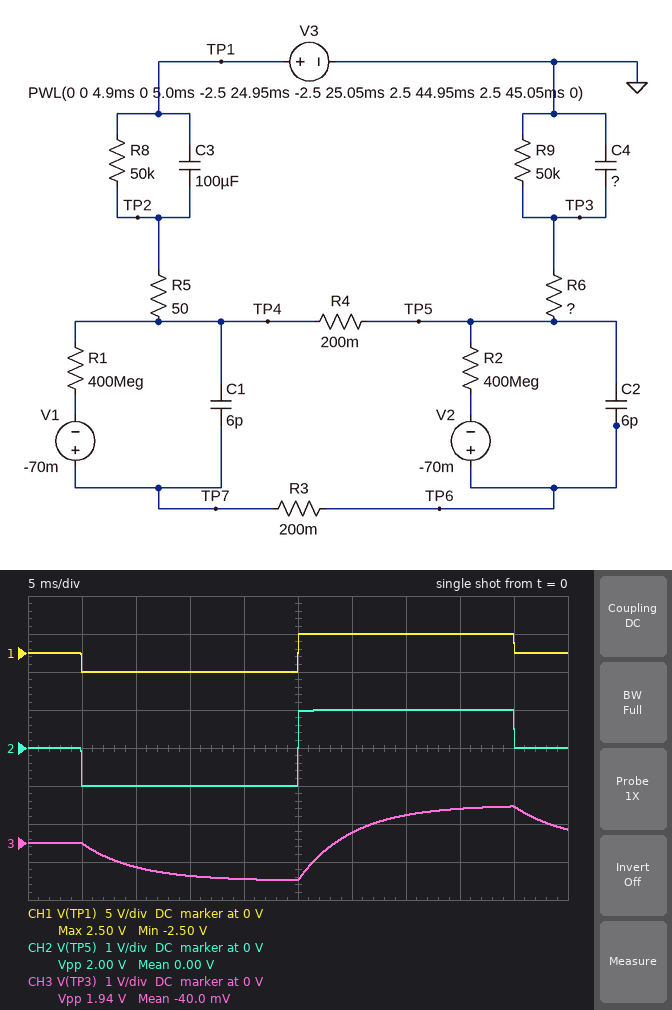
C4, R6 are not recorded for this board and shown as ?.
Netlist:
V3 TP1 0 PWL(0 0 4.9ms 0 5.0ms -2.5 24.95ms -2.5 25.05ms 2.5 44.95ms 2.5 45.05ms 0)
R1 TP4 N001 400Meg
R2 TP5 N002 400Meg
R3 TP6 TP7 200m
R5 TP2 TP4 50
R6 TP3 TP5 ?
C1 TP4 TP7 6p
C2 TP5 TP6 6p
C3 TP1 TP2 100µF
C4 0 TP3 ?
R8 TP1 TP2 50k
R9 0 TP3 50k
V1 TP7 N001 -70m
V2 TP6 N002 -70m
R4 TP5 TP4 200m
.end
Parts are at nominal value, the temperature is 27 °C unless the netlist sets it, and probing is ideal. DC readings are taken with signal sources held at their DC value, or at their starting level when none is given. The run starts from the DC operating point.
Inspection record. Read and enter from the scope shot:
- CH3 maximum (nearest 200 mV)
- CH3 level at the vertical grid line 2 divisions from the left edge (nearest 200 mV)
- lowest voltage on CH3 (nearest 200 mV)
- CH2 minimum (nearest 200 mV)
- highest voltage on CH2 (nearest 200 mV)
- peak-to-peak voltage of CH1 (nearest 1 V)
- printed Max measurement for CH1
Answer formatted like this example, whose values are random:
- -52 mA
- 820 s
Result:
- 1.0 V
- -600 mV
- -1.0 V
- -1.0 V
- 1.0 V
- 5 V
- 2.50 V
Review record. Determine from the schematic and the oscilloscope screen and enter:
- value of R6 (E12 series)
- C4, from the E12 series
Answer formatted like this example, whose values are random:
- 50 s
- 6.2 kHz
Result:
- 33 Ω
- 150 µF
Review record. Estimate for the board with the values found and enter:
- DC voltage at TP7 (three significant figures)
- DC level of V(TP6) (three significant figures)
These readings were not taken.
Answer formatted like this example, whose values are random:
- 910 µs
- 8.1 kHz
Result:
- -70.0 mV
- -70.0 mV
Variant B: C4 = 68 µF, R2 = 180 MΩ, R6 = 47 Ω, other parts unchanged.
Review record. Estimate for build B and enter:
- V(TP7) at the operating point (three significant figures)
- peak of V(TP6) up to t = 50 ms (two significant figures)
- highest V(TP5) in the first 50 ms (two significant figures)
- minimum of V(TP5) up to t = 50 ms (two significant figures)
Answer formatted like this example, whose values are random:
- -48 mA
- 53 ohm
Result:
- -70.0 mV
- 1.4 V
- 1.5 V
- -1.5 V
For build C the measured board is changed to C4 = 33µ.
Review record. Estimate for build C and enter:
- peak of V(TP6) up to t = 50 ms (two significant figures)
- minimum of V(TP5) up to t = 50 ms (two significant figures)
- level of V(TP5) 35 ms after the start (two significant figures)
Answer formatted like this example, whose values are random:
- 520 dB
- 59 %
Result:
- 1.8 V
- -1.9 V
- 1.9 V
